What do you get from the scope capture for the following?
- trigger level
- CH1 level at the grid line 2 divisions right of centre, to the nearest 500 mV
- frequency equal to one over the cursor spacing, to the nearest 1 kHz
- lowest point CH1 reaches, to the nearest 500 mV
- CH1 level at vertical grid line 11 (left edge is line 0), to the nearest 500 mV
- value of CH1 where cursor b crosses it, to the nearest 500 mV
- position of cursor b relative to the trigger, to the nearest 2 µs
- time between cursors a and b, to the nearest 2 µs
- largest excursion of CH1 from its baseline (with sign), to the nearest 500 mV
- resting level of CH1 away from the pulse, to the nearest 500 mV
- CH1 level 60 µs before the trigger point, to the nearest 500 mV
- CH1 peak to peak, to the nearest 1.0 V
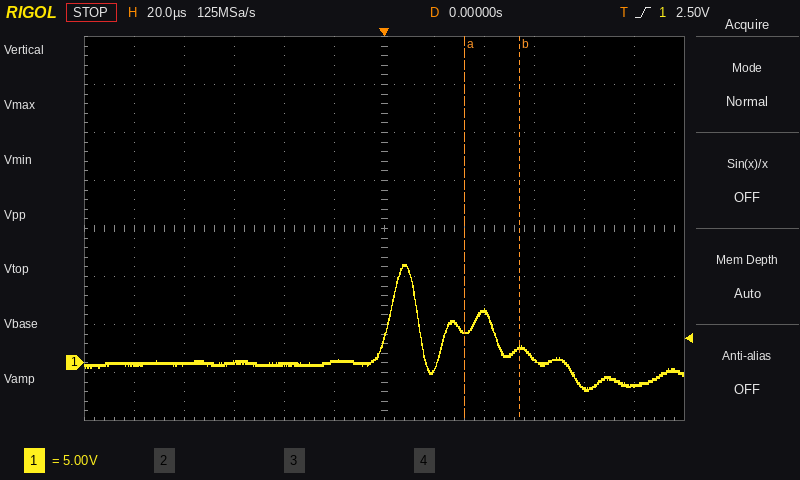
2.50 V
5.5 V
45 kHz
-3.0 V
-2.5 V
1.5 V
+54 µs
22 µs
+10.5 V
0.0 V
0.0 V
13.0 V
